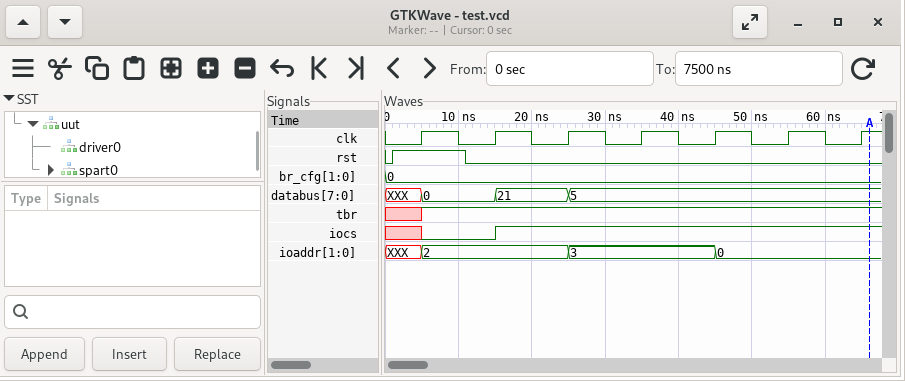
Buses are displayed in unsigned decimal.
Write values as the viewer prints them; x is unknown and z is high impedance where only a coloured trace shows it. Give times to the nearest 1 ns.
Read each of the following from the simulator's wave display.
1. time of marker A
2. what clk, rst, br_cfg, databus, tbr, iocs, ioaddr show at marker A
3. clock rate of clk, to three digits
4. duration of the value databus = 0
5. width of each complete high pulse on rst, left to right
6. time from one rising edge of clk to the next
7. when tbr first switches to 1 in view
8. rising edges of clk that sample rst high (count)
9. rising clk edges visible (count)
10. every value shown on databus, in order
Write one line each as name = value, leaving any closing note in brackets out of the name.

time of marker A = 66 ns
what clk, rst, br_cfg, databus, tbr, iocs, ioaddr show at marker A = clk=1, rst=0, br_cfg=0, databus=5, tbr=1, iocs=1, ioaddr=0
clock rate of clk, to three digits = 100 MHz
duration of the value databus = 0 = 10 ns
width of each complete high pulse on rst, left to right = 10 ns
time from one rising edge of clk to the next = 10 ns
when tbr first switches to 1 in view = 5 ns
rising edges of clk that sample rst high = 1
rising clk edges visible = 7
every value shown on databus, in order = XXX, 0, 21, 5
